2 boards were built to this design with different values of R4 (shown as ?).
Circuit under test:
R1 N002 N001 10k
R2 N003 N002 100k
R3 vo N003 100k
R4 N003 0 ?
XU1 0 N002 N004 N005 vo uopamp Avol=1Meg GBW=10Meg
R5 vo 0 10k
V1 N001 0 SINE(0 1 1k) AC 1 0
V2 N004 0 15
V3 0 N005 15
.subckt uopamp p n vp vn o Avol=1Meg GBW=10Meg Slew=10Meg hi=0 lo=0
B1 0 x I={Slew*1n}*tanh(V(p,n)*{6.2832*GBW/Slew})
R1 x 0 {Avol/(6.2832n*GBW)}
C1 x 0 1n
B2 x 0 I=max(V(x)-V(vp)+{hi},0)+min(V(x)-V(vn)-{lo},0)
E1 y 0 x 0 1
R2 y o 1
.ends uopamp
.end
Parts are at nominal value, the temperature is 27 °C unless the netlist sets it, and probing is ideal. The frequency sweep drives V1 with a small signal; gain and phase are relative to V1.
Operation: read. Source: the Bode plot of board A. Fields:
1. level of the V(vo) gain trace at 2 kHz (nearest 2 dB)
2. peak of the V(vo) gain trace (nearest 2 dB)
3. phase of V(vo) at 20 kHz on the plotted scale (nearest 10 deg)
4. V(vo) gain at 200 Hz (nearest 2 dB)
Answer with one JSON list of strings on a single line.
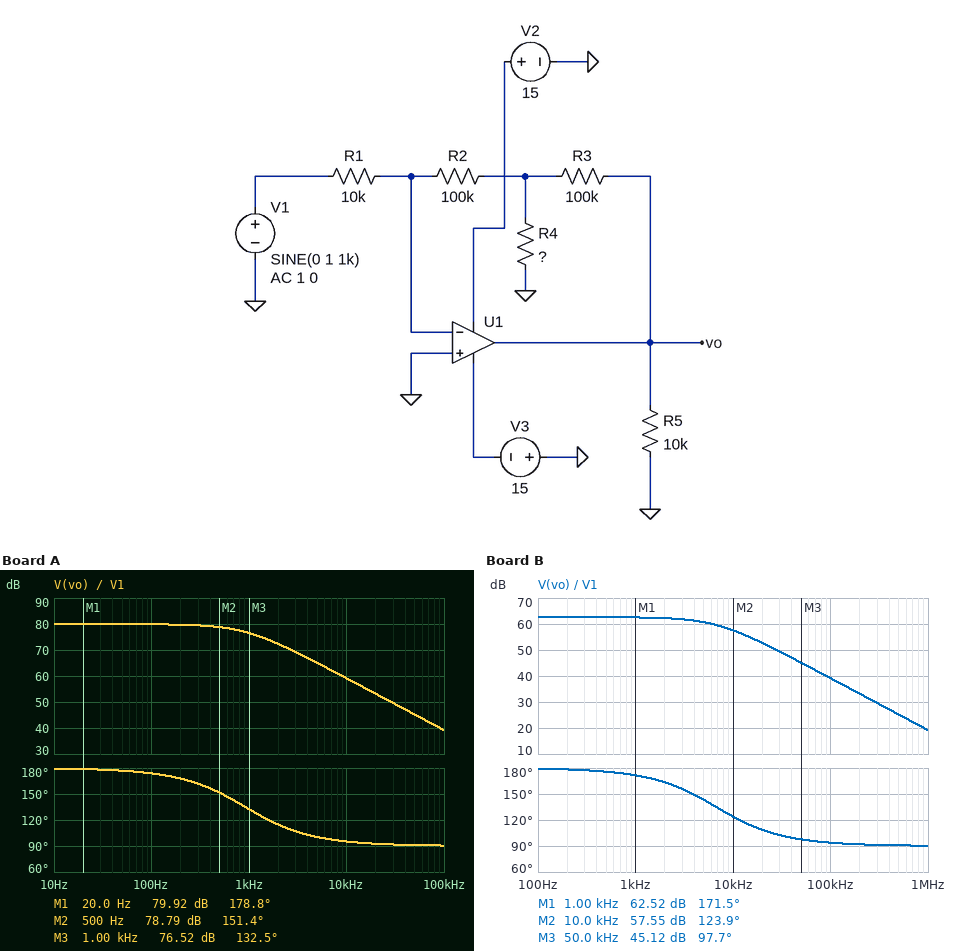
["72 dB", "80 dB", "90 deg", "80 dB"]
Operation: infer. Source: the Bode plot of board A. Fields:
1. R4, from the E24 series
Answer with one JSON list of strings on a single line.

["100 Ω"]
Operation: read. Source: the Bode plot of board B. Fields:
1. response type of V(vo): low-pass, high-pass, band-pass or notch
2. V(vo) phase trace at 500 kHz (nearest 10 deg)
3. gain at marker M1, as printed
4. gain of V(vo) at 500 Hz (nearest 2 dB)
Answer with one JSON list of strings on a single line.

["low-pass", "90 deg", "62.52 dB", "62 dB"]
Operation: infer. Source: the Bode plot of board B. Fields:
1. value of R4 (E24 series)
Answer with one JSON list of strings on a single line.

["750 Ω"]
